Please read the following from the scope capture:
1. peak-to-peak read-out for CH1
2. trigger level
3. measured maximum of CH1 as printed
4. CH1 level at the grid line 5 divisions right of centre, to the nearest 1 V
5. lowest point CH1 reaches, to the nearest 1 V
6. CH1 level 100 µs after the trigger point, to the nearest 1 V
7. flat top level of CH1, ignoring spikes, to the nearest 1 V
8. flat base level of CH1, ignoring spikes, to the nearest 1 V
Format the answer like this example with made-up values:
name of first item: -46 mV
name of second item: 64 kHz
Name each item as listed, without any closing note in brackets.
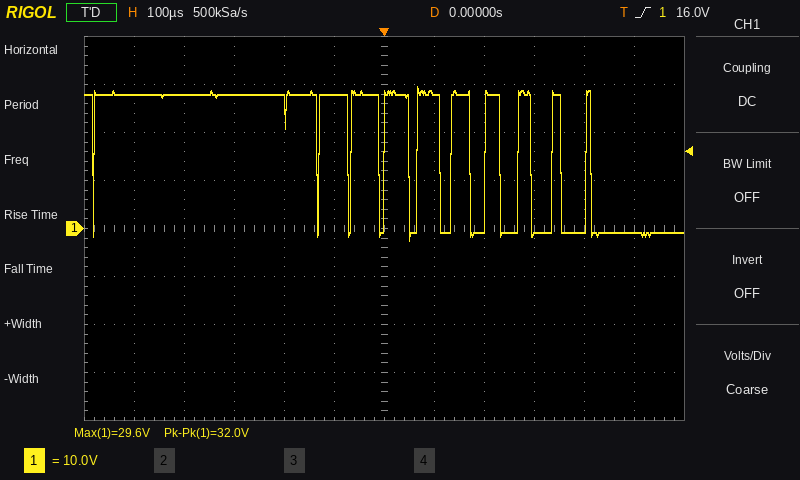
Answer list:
peak-to-peak read-out for CH1: 32.0 V
trigger level: 16.0 V
measured maximum of CH1 as printed: 29.6 V
CH1 level at the grid line 5 divisions right of centre, to the nearest 1 V: -1 V
lowest point CH1 reaches, to the nearest 1 V: -2 V
CH1 level 100 µs after the trigger point, to the nearest 1 V: 28 V
flat top level of CH1, ignoring spikes, to the nearest 1 V: 28 V
flat base level of CH1, ignoring spikes, to the nearest 1 V: -1 V
